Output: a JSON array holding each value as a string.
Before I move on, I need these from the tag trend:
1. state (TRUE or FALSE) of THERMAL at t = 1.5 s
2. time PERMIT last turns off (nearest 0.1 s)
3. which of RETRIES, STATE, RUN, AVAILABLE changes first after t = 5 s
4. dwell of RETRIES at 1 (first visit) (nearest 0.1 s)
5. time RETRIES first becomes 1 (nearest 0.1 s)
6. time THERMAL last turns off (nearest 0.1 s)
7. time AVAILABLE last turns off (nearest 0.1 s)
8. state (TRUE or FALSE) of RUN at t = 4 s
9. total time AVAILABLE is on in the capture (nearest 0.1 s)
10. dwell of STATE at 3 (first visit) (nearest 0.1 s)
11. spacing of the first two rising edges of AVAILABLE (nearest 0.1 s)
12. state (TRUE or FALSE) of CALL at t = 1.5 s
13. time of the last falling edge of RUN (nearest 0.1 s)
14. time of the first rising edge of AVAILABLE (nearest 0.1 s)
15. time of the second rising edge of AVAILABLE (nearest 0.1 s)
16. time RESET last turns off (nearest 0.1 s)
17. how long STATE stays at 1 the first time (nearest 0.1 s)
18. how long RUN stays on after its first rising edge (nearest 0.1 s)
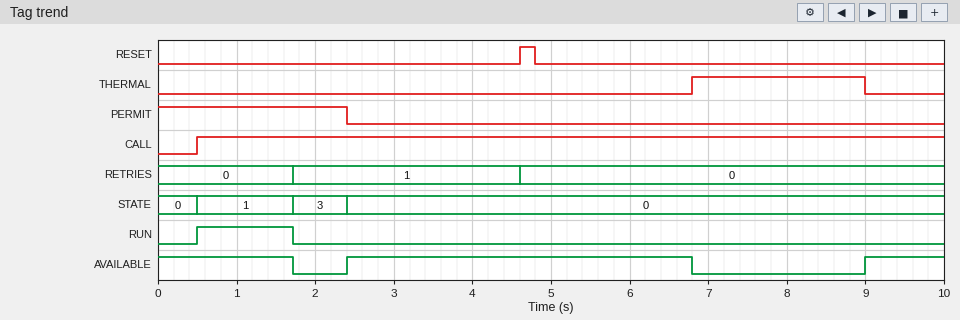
["FALSE", "2.4 s", "AVAILABLE", "2.9 s", "1.7 s", "9.0 s", "6.8 s", "FALSE", "7.1 s", "0.7 s", "6.6 s", "TRUE", "1.7 s", "2.4 s", "9.0 s", "4.8 s", "1.2 s", "1.2 s"]
